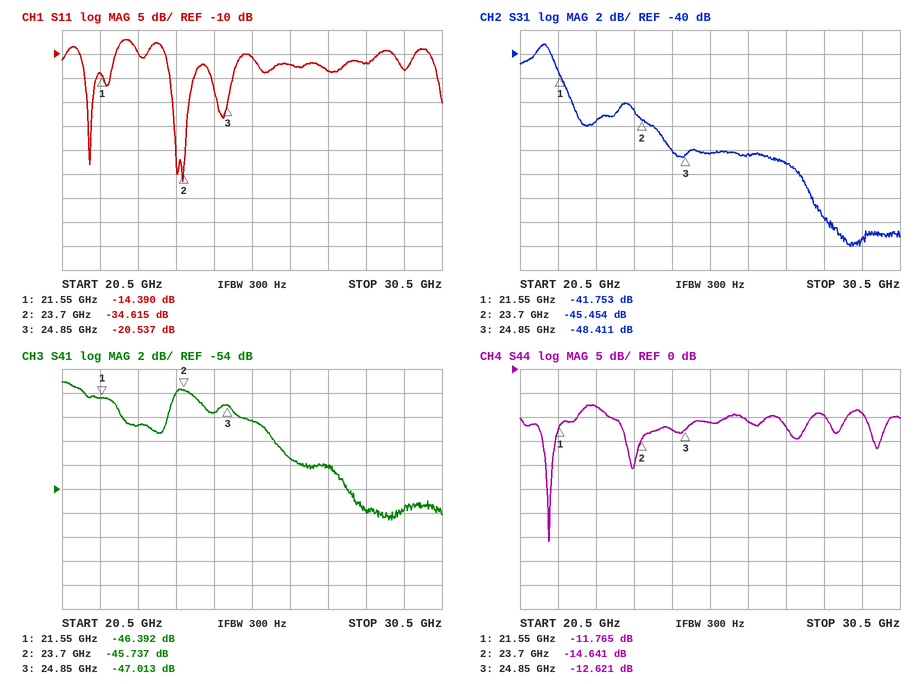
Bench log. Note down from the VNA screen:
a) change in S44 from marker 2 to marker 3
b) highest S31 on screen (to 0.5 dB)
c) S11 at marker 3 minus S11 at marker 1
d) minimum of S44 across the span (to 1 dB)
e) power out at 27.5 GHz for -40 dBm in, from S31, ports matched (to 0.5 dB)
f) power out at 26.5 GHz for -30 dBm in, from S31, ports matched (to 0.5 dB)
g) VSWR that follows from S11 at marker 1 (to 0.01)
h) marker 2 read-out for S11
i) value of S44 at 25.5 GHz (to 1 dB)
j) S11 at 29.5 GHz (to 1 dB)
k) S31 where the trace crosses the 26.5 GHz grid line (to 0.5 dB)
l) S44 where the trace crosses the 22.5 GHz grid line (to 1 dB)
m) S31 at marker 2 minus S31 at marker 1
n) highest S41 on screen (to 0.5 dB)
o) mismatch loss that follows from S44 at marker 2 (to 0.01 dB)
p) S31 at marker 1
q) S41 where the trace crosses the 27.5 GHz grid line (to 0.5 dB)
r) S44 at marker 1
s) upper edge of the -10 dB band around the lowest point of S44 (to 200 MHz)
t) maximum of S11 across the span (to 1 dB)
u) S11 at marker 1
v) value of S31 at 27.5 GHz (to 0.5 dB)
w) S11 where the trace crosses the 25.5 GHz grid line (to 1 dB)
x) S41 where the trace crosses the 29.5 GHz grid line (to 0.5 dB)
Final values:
2.020 dB
-39.0 dB
-6.147 dB
-36 dB
-89.0 dBm
-78.5 dBm
1.47
-34.615 dB
-11 dB
-13 dB
-48.5 dB
-8 dB
-3.701 dB
-45.0 dB
0.15 dB
-41.753 dB
-52.0 dB
-11.765 dB
22.0 GHz
-7 dB
-14.390 dB
-49.0 dB
-11 dB
-55.5 dB
